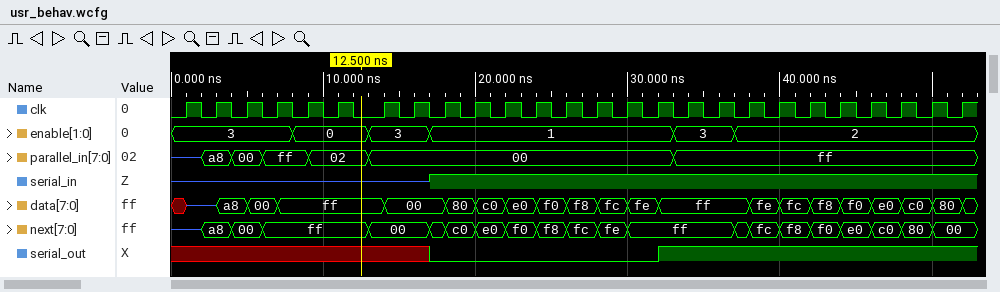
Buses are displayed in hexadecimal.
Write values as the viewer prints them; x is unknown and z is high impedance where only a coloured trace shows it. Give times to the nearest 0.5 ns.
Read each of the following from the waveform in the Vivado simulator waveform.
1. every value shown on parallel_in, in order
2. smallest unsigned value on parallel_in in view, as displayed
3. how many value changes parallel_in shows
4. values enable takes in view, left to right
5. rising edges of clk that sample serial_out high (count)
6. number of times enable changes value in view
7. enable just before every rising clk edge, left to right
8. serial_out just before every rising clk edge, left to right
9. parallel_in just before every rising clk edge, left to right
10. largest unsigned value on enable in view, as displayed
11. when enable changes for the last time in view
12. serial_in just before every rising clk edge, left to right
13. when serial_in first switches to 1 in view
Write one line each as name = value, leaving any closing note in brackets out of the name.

every value shown on parallel_in, in order = z, a8, 00, ff, 02, 00, ff
smallest unsigned value on parallel_in in view, as displayed = 00
how many value changes parallel_in shows = 6
values enable takes in view, left to right = 3, 0, 3, 1, 3, 2
rising edges of clk that sample serial_out high = 10
number of times enable changes value in view = 5
enable just before every rising clk edge, left to right = 3, 3, 3, 3, 0, 0, 3, 3, 1, 1, 1, 1, 1, 1, 1, 1, 3, 3, 2, 2, 2, 2, 2, 2, 2, 2
serial_out just before every rising clk edge, left to right = x x x x x x x x 0 0 0 0 0 0 0 0 1 1 1 1 1 1 1 1 1 1
parallel_in just before every rising clk edge, left to right = z, a8, 00, ff, ff, 02, 00, 00, 00, 00, 00, 00, 00, 00, 00, 00, ff, ff, ff, ff, ff, ff, ff, ff, ff, ff
largest unsigned value on enable in view, as displayed = 3
when enable changes for the last time in view = 37 ns
serial_in just before every rising clk edge, left to right = z z z z z z z z 1 1 1 1 1 1 1 1 1 1 1 1 1 1 1 1 1 1
when serial_in first switches to 1 in view = 17 ns
